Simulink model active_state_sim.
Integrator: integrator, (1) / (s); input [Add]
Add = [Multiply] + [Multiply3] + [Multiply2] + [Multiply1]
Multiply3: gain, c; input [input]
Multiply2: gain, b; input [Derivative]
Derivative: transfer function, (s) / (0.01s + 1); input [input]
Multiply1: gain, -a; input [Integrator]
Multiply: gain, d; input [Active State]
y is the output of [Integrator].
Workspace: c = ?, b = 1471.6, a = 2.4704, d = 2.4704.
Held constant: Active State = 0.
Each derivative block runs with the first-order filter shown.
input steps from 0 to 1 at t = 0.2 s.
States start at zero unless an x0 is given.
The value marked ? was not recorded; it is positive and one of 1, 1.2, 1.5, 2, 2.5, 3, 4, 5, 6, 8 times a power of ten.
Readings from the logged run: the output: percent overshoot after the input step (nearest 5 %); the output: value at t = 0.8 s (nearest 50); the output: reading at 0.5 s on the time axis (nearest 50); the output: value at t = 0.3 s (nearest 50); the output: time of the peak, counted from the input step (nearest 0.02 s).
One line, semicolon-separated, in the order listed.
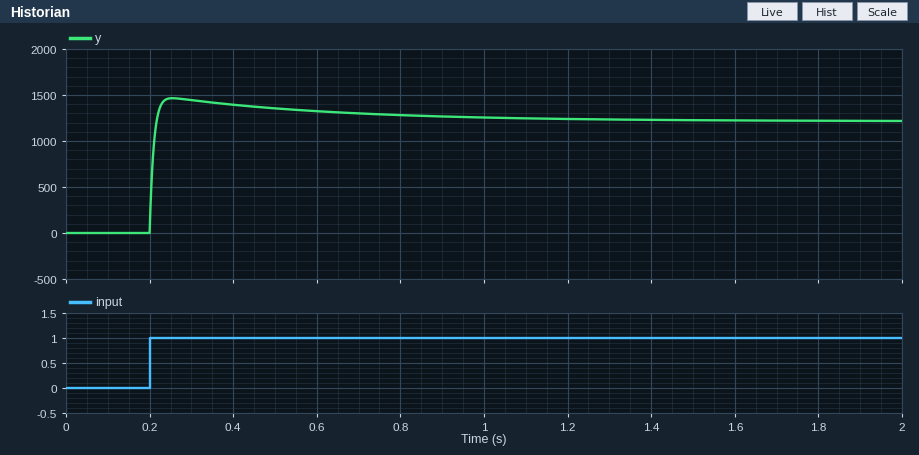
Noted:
20 %; 1300; 1350; 1450; 0.06 s
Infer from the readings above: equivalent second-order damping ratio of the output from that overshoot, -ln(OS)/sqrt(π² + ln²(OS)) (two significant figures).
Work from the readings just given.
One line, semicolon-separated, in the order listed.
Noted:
0.46
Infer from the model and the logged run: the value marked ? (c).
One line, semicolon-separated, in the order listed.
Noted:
3000
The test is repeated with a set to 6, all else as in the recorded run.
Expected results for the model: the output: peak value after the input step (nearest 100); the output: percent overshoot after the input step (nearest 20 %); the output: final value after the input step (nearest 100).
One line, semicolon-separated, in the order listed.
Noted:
1300; 160 %; 500
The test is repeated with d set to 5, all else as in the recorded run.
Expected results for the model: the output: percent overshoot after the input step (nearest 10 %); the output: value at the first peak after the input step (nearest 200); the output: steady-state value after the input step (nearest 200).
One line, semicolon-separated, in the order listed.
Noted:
20 %; 1400; 1200
